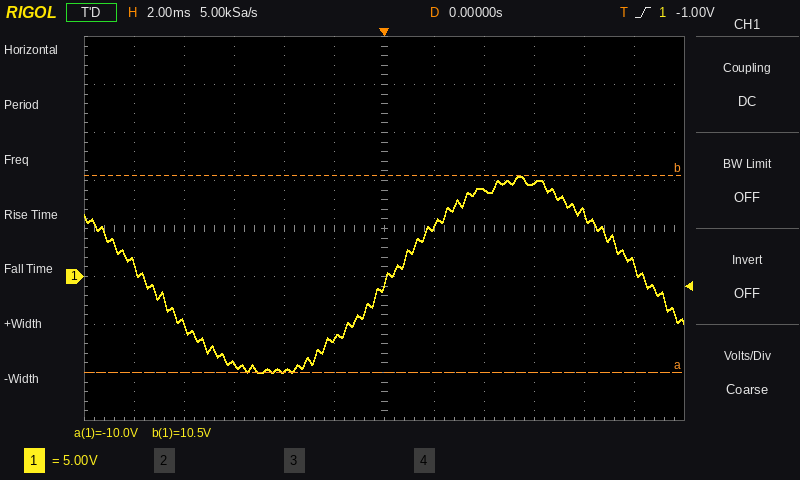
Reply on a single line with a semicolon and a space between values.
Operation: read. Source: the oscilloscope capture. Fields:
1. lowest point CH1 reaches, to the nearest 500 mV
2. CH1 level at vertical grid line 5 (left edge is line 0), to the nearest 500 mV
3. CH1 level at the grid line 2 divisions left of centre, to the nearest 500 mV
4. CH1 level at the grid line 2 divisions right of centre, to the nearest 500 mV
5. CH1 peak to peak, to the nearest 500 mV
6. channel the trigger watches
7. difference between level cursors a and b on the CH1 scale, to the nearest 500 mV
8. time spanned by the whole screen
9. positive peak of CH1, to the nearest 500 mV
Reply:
-10.0 V; -6.5 V; -10.0 V; 9.0 V; 20.5 V; CH1; 20.5 V; 24 ms; 10.5 V
